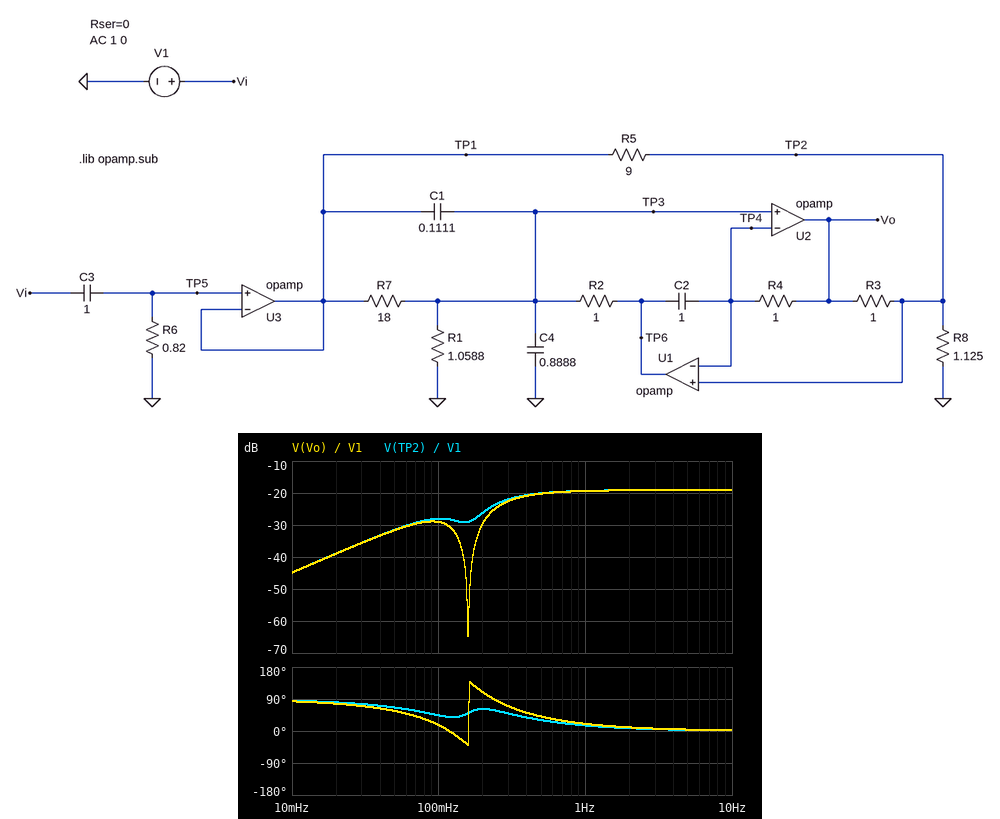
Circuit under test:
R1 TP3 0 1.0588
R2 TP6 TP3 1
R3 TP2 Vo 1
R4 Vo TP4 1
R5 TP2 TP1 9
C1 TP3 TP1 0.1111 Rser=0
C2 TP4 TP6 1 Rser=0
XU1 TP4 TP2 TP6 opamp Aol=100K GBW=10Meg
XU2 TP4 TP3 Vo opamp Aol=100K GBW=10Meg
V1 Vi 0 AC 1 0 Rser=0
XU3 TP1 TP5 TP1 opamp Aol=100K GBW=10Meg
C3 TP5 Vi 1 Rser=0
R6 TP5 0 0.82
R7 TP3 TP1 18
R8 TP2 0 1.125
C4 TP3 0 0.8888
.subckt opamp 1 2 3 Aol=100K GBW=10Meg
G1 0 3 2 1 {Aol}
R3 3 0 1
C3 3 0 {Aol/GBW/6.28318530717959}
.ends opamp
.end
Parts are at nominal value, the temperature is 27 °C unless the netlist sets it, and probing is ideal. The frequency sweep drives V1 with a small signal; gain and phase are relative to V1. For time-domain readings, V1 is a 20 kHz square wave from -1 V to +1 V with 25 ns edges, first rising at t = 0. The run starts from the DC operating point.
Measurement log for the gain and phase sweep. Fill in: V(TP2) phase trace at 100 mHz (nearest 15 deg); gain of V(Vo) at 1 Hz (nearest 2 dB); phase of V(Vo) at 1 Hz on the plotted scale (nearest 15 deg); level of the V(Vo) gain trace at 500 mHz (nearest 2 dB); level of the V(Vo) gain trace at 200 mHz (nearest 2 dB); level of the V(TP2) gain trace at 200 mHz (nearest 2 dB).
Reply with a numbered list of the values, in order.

1. 45 deg
2. -20 dB
3. 15 deg
4. -20 dB
5. -30 dB
6. -26 dB
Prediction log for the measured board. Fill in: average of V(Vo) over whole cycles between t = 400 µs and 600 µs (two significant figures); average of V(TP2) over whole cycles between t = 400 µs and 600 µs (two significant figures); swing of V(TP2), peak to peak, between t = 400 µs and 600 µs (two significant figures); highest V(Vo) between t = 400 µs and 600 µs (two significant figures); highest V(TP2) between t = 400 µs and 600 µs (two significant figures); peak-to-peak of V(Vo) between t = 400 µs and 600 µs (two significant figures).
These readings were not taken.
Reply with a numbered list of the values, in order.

1. 110 mV
2. 110 mV
3. 220 mV
4. 220 mV
5. 220 mV
6. 220 mV
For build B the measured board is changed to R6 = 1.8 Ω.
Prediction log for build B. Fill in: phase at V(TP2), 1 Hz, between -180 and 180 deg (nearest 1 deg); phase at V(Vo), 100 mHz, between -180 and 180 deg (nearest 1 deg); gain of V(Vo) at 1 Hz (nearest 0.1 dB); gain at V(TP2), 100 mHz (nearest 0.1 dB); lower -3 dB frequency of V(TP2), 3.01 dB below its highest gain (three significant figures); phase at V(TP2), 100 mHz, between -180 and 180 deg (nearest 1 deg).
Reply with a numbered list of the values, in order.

1. 10 deg
2. -5 deg
3. -19.2 dB
4. -23.7 dB
5. 241 mHz
6. 23 deg
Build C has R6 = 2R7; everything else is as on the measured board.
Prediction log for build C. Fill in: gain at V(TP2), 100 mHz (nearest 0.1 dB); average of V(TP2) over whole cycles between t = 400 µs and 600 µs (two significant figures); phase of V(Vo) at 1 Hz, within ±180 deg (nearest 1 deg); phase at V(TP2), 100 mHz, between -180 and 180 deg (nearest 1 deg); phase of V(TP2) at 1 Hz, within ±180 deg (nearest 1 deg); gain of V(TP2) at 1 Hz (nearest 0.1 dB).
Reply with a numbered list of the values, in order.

1. -22.5 dB
2. 110 mV
3. 13 deg
4. 12 deg
5. 8 deg
6. -19.2 dB
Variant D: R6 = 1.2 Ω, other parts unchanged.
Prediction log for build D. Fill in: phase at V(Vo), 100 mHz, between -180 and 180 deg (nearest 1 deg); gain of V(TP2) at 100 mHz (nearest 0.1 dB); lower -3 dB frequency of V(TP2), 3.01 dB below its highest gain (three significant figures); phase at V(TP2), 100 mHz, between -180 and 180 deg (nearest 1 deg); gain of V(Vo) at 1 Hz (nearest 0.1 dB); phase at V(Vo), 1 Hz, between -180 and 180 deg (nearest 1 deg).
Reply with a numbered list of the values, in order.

1. 7 deg
2. -25.6 dB
3. 259 mHz
4. 34 deg
5. -19.3 dB
6. 17 deg
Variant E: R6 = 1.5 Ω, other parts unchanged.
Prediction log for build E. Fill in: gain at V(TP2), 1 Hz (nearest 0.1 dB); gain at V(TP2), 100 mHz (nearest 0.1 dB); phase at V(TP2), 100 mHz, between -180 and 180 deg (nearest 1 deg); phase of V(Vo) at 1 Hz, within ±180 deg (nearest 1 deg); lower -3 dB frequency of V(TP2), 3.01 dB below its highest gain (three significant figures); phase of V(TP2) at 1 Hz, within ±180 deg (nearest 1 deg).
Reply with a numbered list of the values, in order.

1. -19.2 dB
2. -24.5 dB
3. 28 deg
4. 15 deg
5. 248 mHz
6. 11 deg
